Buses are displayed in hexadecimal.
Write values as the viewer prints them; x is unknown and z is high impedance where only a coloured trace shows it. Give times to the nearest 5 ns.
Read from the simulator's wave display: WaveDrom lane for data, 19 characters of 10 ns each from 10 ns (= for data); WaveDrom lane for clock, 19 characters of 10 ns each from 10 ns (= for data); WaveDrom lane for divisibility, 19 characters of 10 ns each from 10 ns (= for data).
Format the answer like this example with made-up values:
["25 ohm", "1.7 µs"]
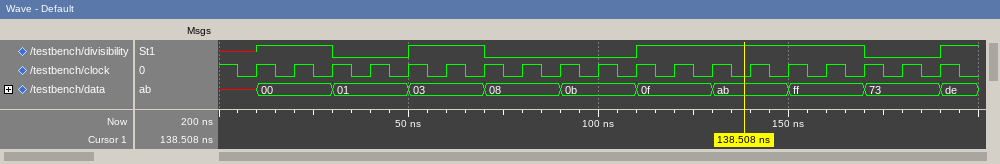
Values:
["{name: 'data', wave: '=.=.=.=.=.=.=.=.=.=', data: '00 01 03 08 0b 0f ab ff 73 de'}", "{name: 'clock', wave: 'p..................'}", "{name: 'divisibility', wave: '1.0.1.0...1.....0.1'}"]
